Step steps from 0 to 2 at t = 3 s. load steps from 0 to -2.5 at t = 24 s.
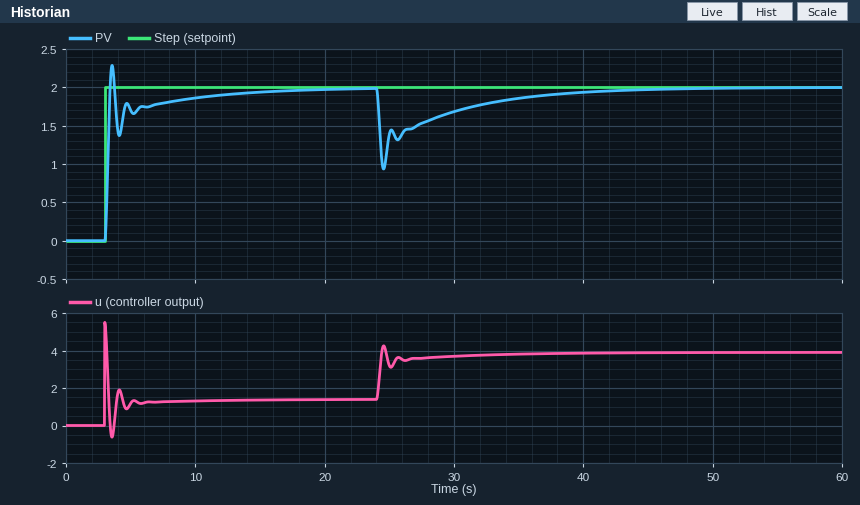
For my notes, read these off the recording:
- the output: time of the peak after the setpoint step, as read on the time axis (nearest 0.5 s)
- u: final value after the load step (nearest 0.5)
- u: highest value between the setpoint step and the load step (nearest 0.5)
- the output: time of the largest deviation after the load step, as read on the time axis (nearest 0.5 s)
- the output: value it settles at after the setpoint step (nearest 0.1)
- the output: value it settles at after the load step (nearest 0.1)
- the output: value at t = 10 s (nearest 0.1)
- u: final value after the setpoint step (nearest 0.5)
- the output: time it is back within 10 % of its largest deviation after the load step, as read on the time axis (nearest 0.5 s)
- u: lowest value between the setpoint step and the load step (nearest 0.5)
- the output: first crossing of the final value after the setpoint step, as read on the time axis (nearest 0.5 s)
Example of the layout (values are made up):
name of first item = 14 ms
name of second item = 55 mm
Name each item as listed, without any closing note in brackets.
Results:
the output: time of the peak after the setpoint step, as read on the time axis = 3.5 s
u: final value after the load step = 4.0
u: highest value between the setpoint step and the load step = 5.5
the output: time of the largest deviation after the load step, as read on the time axis = 24.5 s
the output: value it settles at after the setpoint step = 2.0
the output: value it settles at after the load step = 2.0
the output: value at t = 10 s = 1.9
u: final value after the setpoint step = 1.5
the output: time it is back within 10 % of its largest deviation after the load step, as read on the time axis = 37.0 s
u: lowest value between the setpoint step and the load step = -0.5
the output: first crossing of the final value after the setpoint step, as read on the time axis = 3.5 s
